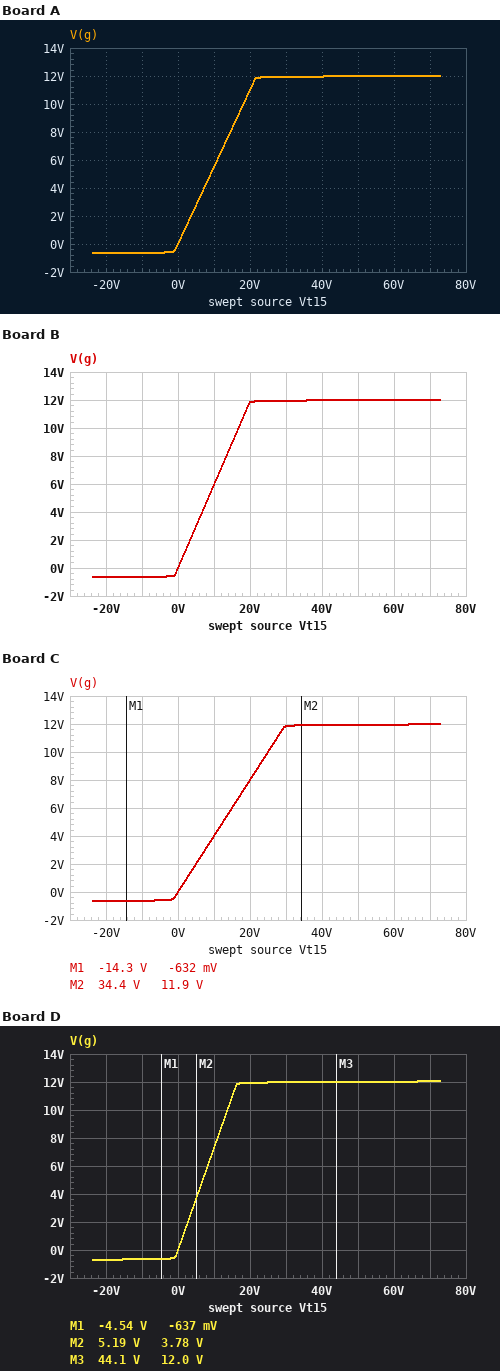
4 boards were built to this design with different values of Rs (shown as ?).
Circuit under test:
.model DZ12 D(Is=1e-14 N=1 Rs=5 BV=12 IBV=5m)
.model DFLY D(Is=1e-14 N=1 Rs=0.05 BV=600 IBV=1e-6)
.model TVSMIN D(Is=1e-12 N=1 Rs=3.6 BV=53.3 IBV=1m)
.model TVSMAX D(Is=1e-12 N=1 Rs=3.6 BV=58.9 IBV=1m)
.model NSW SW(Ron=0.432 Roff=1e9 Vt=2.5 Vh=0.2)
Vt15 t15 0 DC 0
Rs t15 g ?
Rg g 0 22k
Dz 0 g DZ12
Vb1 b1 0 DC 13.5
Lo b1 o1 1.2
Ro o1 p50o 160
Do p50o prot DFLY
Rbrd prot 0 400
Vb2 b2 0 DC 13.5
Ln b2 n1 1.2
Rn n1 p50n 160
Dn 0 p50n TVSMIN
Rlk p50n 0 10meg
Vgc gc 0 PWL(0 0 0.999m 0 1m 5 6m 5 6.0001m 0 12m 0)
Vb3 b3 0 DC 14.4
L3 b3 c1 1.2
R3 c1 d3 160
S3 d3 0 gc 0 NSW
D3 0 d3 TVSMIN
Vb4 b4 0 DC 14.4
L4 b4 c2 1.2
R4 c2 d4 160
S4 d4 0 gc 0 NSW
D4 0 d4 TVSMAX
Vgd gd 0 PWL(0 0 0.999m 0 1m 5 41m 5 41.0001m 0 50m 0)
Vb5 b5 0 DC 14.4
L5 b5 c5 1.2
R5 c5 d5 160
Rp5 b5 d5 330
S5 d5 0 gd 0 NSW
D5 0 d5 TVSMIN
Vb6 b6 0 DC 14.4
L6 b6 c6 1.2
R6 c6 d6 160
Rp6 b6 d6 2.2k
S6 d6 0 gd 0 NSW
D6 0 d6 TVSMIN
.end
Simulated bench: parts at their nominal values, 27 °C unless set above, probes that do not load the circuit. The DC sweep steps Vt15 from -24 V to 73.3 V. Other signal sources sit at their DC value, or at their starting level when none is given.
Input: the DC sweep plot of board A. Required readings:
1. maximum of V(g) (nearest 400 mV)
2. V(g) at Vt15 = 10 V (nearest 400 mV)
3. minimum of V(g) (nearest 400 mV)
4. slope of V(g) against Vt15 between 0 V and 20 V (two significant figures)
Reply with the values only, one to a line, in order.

12.0 V
5.6 V
-800 mV
0.55 V/V
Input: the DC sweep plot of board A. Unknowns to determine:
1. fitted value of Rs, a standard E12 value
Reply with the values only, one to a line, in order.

18 kΩ
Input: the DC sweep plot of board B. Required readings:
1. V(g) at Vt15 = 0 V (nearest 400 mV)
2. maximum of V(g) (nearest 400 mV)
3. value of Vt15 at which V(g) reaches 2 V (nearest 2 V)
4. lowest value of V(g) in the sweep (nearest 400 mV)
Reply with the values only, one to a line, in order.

0 V
12.0 V
4 V
-800 mV
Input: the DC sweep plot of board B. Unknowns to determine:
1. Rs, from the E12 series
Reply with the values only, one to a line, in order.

15 kΩ
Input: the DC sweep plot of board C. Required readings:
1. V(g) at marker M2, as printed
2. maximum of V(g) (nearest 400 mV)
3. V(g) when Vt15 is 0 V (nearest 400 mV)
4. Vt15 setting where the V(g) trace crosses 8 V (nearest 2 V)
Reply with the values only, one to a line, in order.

11.9 V
12.0 V
0 V
20 V
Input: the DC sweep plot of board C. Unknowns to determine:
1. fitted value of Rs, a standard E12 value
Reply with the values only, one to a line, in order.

33 kΩ
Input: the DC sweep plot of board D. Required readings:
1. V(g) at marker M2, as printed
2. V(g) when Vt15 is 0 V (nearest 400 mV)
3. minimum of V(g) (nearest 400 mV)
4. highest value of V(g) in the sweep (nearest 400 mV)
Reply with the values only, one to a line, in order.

3.78 V
0 V
-800 mV
12.0 V
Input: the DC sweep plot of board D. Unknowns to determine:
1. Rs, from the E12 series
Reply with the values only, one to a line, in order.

8.2 kΩ
